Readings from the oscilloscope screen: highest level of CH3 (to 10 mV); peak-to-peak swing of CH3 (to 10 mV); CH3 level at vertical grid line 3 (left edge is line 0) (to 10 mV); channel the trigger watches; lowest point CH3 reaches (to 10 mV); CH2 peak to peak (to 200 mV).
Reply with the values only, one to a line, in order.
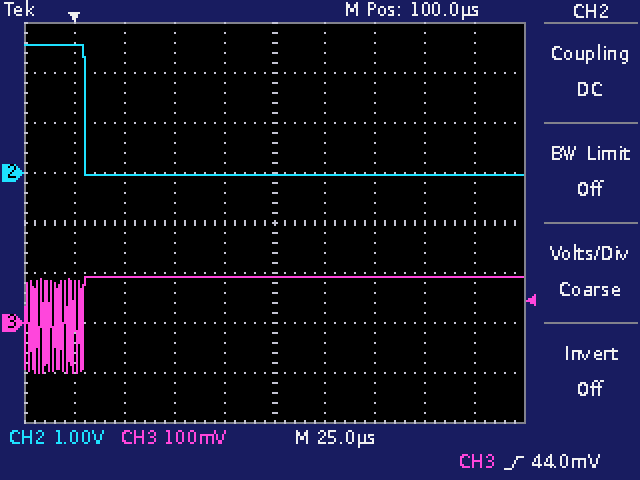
90 mV
190 mV
90 mV
CH3
-100 mV
2.6 V
